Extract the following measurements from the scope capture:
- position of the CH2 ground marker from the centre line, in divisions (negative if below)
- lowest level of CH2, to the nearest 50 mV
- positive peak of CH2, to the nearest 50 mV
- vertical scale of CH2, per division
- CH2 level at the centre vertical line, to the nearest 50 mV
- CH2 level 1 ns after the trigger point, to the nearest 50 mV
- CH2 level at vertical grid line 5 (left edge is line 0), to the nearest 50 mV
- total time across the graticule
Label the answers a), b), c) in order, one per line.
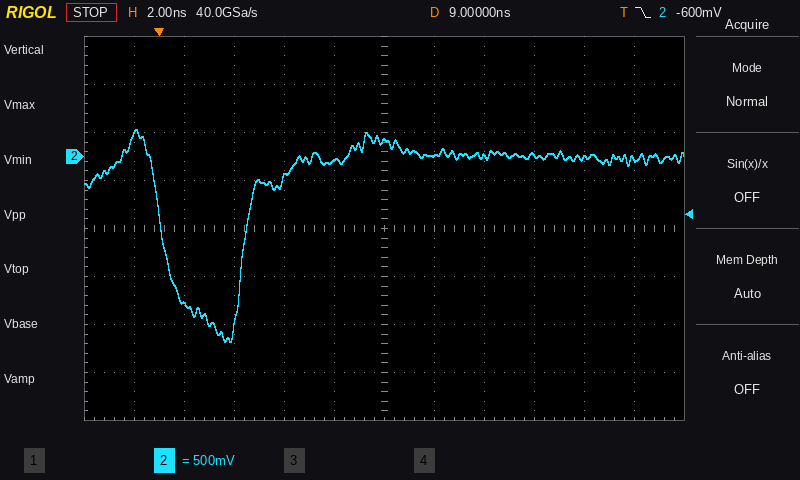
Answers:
a) +1.5 div
b) -1.95 V
c) 300 mV
d) 500 mV
e) 150 mV
f) -1.55 V
g) -50 mV
h) 24 ns
